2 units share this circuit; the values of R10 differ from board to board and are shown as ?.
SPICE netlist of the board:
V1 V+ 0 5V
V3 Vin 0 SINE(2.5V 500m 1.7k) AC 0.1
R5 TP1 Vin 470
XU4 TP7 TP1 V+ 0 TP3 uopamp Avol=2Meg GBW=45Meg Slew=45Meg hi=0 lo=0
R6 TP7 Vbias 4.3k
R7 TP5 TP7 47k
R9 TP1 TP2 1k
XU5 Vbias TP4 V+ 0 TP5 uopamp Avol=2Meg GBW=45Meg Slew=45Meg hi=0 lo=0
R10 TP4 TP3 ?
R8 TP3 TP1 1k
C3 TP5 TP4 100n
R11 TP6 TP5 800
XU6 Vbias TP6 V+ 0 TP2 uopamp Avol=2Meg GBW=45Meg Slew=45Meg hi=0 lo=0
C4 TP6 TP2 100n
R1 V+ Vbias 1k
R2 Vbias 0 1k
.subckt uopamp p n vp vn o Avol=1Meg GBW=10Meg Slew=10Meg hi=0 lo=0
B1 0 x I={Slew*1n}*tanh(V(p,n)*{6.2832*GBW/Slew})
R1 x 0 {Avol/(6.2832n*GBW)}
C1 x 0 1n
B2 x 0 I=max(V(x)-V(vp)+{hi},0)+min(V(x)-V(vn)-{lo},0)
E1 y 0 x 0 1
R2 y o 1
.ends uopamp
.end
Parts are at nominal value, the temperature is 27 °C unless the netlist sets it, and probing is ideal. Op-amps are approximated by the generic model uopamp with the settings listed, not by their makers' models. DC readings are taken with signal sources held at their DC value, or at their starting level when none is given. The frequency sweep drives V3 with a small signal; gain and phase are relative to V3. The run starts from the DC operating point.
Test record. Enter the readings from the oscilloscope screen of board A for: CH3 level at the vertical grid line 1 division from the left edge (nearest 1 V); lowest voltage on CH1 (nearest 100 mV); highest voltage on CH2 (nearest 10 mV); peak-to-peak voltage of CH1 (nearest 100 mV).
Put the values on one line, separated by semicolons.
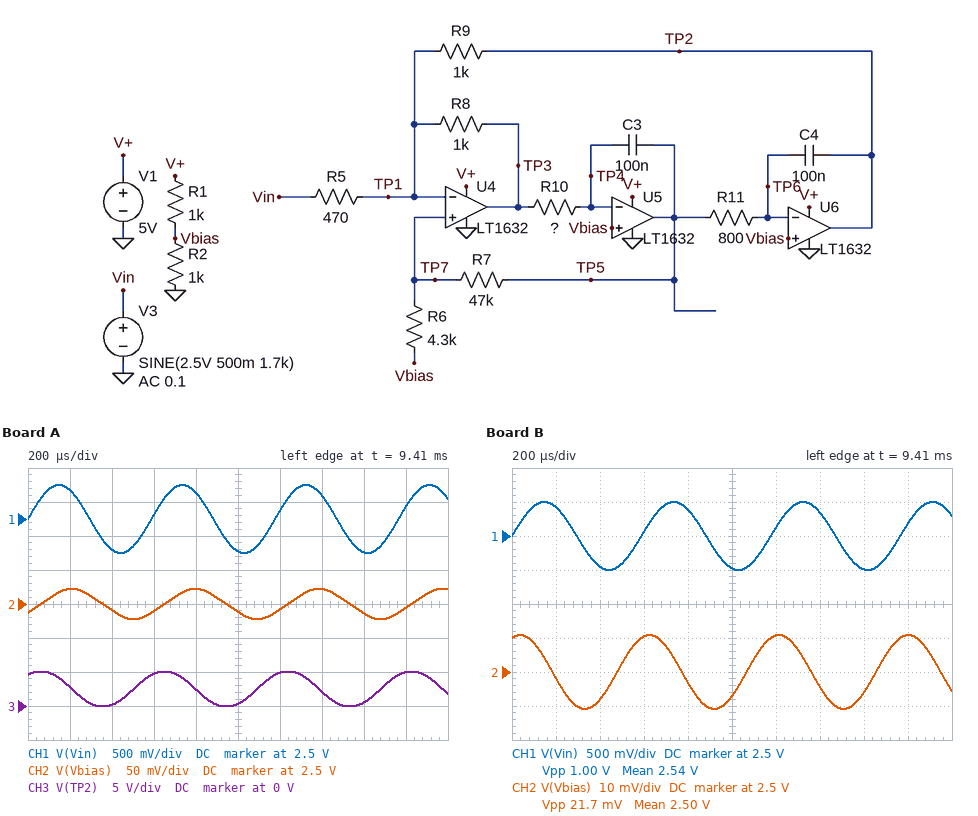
3 V; 2.0 V; 2.52 V; 1.0 V
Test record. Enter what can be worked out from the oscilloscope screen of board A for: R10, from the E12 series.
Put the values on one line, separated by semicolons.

1.2 kΩ
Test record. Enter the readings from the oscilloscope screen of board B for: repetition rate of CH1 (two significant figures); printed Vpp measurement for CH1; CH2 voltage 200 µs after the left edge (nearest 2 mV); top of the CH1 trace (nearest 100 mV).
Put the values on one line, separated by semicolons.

1.7 kHz; 1.00 V; 2.498 V; 3.0 V
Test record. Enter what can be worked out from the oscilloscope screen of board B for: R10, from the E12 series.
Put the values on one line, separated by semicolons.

270 Ω
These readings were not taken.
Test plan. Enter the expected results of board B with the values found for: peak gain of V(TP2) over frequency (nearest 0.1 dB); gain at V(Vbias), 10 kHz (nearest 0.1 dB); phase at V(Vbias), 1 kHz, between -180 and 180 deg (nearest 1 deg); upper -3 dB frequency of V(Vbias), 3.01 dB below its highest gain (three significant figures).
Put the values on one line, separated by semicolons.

11.0 dB; -37.4 dB; 79 deg; 4.67 kHz
